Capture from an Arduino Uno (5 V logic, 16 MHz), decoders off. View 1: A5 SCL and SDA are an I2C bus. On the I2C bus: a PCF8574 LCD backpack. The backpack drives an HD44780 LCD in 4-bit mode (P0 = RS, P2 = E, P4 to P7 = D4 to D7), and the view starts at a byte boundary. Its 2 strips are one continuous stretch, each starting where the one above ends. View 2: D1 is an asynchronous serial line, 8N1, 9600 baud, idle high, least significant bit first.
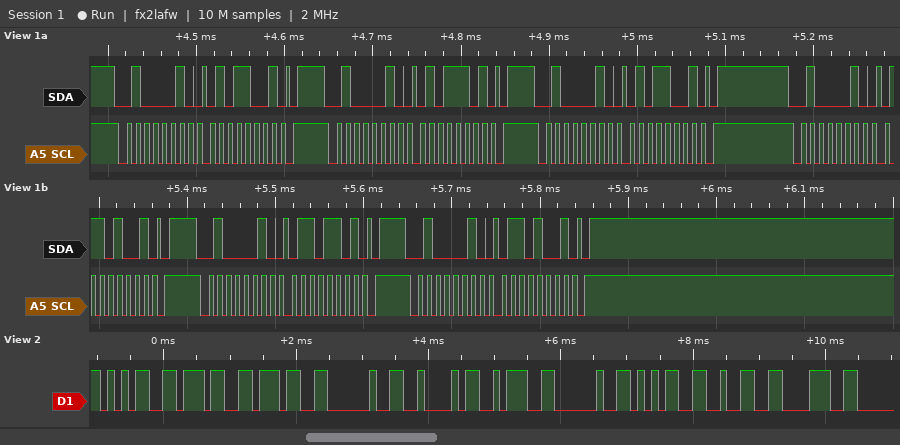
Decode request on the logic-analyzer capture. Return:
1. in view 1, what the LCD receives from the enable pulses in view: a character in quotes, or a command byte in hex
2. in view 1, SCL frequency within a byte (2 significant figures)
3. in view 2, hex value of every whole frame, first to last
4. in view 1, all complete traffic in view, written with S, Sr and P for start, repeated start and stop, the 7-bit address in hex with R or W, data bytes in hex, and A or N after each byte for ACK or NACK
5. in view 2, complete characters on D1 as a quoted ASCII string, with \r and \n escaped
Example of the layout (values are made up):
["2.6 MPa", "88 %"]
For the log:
["'V'", "100 kHz", "0x35 0x37 0x37 0x20 0x42 0x3A 0x20 0x35 0x32 0x38", "S 21W A 59 A P S 21W A 5D A P S 21W A 59 A P S 21W A 69 A P S 21W A 6D A P S 21W A 69 A P", "\"577 B: 528\""]
